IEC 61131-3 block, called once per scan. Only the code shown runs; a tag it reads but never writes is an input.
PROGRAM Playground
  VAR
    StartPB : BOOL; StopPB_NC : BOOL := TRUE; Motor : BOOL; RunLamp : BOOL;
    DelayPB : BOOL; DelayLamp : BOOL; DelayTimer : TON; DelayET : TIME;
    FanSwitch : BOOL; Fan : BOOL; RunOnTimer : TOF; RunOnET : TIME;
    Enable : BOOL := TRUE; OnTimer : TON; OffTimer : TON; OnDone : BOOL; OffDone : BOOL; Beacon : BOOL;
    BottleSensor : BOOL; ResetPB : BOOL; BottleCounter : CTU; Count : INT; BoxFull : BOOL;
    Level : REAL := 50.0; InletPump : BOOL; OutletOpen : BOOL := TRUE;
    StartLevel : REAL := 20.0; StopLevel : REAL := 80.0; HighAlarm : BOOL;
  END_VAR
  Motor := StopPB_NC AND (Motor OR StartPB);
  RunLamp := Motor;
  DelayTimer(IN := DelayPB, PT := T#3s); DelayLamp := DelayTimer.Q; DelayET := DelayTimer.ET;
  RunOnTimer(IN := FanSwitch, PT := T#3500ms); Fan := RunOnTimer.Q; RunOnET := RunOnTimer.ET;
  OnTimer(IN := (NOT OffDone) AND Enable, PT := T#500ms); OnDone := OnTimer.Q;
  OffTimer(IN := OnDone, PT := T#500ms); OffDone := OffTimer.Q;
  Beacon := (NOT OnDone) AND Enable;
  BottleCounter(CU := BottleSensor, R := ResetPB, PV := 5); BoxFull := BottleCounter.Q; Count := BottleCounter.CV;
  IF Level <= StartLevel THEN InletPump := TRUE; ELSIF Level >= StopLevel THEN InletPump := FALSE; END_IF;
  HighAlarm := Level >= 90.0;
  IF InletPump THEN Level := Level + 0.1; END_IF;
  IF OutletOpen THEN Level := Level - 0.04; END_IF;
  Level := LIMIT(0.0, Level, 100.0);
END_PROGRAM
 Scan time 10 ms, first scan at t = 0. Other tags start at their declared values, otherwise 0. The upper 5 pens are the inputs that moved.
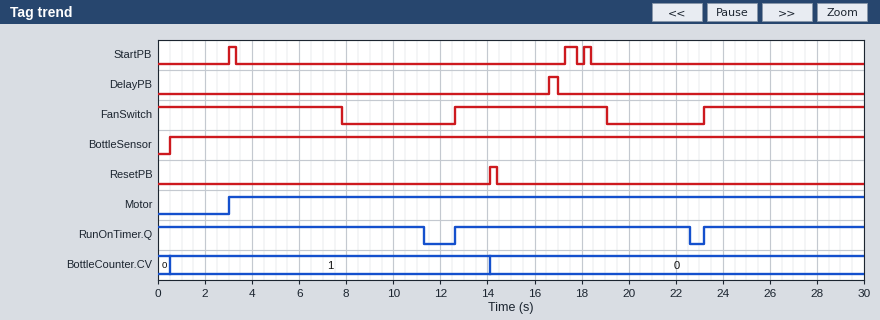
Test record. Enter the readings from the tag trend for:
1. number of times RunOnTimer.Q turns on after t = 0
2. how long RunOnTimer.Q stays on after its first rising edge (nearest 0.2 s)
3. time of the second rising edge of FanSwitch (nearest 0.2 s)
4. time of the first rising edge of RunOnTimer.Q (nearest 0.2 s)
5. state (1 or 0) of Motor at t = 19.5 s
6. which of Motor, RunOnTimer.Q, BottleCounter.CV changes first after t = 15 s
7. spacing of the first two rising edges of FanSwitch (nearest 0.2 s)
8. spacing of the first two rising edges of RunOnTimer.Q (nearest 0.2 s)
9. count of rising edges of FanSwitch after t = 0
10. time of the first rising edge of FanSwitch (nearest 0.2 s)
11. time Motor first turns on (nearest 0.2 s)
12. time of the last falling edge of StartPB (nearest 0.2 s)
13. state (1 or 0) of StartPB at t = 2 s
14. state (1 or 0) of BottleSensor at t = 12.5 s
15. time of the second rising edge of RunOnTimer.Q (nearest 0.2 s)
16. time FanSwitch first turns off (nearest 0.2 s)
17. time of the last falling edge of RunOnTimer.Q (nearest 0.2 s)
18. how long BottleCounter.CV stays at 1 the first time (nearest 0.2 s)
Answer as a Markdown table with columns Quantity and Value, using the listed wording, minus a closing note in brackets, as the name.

| Quantity | Value |
|---|---|
| number of times RunOnTimer.Q turns on after t = 0 | 2 |
| how long RunOnTimer.Q stays on after its first rising edge | 10.0 s |
| time of the second rising edge of FanSwitch | 23.2 s |
| time of the first rising edge of RunOnTimer.Q | 12.6 s |
| state (1 or 0) of Motor at t = 19.5 s | 1 |
| which of Motor, RunOnTimer.Q, BottleCounter.CV changes first after t = 15 s | RunOnTimer.Q |
| spacing of the first two rising edges of FanSwitch | 10.6 s |
| spacing of the first two rising edges of RunOnTimer.Q | 10.6 s |
| count of rising edges of FanSwitch after t = 0 | 2 |
| time of the first rising edge of FanSwitch | 12.6 s |
| time Motor first turns on | 3.0 s |
| time of the last falling edge of StartPB | 18.4 s |
| state (1 or 0) of StartPB at t = 2 s | 0 |
| state (1 or 0) of BottleSensor at t = 12.5 s | 1 |
| time of the second rising edge of RunOnTimer.Q | 23.2 s |
| time FanSwitch first turns off | 7.8 s |
| time of the last falling edge of RunOnTimer.Q | 22.6 s |
| how long BottleCounter.CV stays at 1 the first time | 13.6 s |
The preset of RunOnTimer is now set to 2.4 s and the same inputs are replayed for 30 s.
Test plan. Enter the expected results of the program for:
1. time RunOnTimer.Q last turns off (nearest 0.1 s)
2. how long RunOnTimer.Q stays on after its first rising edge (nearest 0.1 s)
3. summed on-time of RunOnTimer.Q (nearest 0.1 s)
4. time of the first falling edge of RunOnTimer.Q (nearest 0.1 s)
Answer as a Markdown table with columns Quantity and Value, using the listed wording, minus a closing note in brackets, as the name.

| Quantity | Value |
|---|---|
| time RunOnTimer.Q last turns off | 21.5 s |
| how long RunOnTimer.Q stays on after its first rising edge | 8.9 s |
| summed on-time of RunOnTimer.Q | 25.9 s |
| time of the first falling edge of RunOnTimer.Q | 10.2 s |
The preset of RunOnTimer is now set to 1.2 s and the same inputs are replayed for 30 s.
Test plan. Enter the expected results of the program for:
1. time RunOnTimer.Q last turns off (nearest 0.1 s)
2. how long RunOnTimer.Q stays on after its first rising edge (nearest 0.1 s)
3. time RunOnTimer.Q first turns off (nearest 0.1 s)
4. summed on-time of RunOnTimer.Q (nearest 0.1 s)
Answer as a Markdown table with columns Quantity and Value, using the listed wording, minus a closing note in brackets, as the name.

| Quantity | Value |
|---|---|
| time RunOnTimer.Q last turns off | 20.3 s |
| how long RunOnTimer.Q stays on after its first rising edge | 7.7 s |
| time RunOnTimer.Q first turns off | 9.0 s |
| summed on-time of RunOnTimer.Q | 23.5 s |
